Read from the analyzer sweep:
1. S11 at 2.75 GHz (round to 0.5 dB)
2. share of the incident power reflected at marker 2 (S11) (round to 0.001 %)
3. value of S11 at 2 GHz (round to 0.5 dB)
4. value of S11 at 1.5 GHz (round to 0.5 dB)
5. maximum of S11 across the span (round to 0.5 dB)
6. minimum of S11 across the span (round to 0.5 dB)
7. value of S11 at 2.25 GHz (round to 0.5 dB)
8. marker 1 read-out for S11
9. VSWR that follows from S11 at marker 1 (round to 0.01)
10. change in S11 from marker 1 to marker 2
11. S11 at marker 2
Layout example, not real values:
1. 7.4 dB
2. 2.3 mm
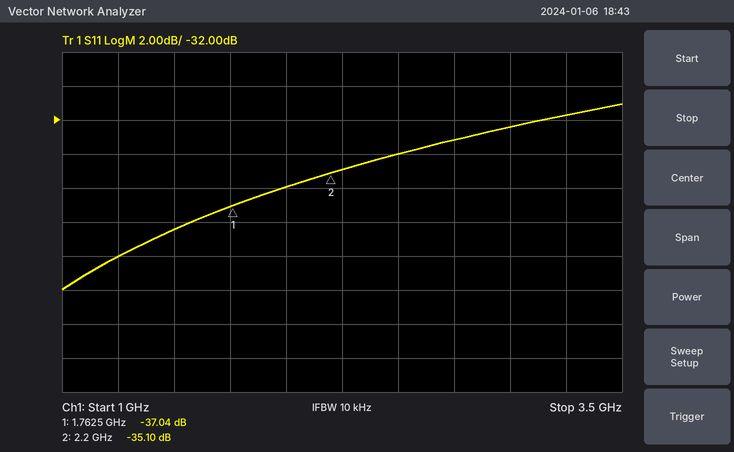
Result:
1. -33.0 dB
2. 0.031 %
3. -36.0 dB
4. -38.5 dB
5. -31.0 dB
6. -42.0 dB
7. -35.0 dB
8. -37.04 dB
9. 1.03
10. 1.94 dB
11. -35.10 dB
